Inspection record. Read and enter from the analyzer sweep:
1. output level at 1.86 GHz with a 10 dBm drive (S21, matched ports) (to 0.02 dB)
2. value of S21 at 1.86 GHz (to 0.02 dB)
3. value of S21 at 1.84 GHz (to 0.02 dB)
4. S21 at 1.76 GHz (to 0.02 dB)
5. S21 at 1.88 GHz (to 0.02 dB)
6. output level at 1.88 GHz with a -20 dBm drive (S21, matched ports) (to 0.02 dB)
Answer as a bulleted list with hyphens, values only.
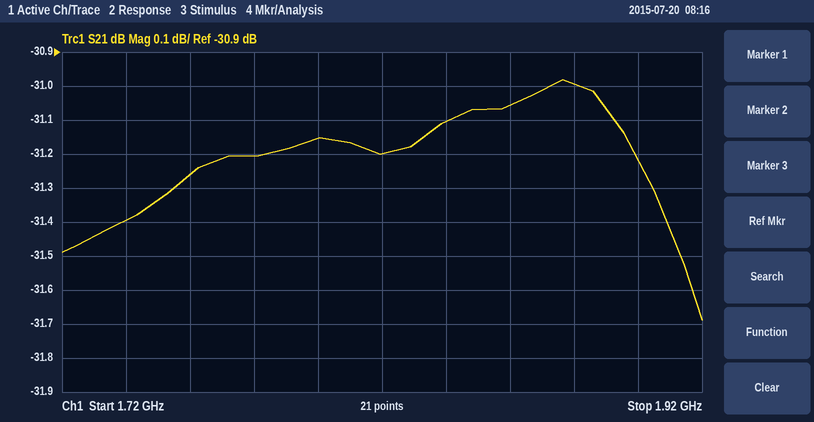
- -21.06 dBm
- -31.06 dB
- -31.10 dB
- -31.26 dB
- -31.00 dB
- -51.00 dBm
